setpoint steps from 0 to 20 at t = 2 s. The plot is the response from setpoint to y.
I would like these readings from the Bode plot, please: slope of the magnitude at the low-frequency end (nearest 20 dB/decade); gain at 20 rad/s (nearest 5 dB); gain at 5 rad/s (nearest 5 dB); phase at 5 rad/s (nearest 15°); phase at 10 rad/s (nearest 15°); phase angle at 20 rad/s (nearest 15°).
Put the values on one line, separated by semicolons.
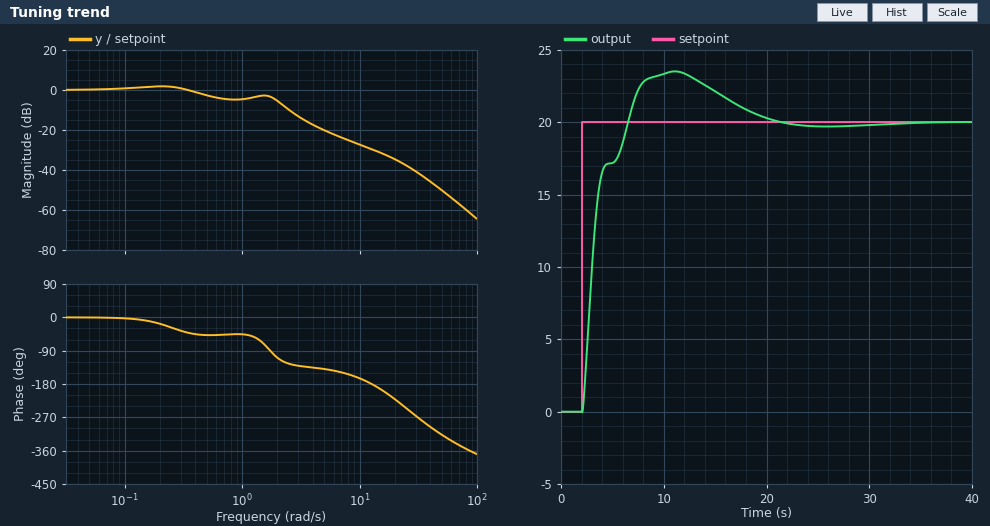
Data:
0 dB/decade; -35 dB; -20 dB; -135°; -165°; -225°
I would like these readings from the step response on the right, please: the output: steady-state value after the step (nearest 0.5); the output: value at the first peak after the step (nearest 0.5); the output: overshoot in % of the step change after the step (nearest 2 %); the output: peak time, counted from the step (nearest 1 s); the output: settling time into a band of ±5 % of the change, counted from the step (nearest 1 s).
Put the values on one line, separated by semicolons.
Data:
20.0; 23.5; 18 %; 9 s; 16 s
